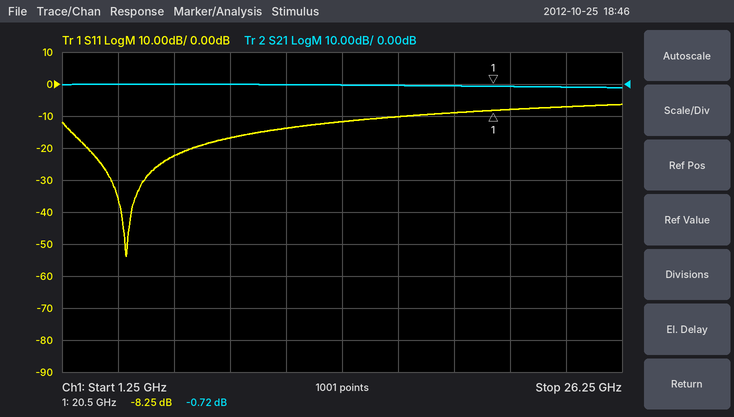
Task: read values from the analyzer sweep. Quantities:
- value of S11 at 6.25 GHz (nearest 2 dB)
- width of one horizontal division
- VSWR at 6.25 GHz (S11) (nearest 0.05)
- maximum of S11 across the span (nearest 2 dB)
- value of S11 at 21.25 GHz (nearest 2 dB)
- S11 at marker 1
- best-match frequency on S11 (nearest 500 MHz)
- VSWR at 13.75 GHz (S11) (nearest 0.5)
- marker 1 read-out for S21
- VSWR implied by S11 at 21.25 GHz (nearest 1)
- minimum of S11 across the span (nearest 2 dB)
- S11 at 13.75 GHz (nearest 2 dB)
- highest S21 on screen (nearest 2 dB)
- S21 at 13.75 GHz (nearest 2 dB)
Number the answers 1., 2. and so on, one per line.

1. -22 dB
2. 2.5 GHz
3. 1.15
4. -6 dB
5. -8 dB
6. -8.25 dB
7. 4.0 GHz
8. 1.5
9. -0.72 dB
10. 2
11. -54 dB
12. -12 dB
13. 0 dB
14. 0 dB
